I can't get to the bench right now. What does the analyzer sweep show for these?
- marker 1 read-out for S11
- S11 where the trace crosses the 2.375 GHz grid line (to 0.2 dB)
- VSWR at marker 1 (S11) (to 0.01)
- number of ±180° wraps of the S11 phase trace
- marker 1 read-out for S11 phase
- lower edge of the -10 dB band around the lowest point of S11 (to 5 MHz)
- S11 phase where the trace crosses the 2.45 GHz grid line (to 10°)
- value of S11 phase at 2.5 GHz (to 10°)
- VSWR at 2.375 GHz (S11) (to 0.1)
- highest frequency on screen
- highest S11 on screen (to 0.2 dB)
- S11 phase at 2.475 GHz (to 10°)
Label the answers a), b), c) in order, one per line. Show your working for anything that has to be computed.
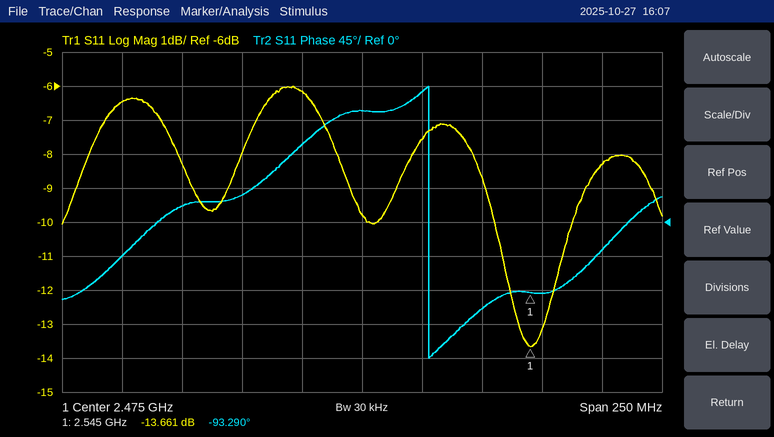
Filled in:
a) -13.661 dB
b) -6.4 dB
c) (1 + 0.2075)/(1 − 0.2075) ≈ 1.52
d) 1
e) -93.290°
f) 2.530 GHz
g) 100°
h) 170°
i) |Γ| = 10^(-6.4/20) = 0.4786; VSWR = (1 + 0.4786)/(1 − 0.4786) ≈ 2.8
j) 2.6 GHz
k) -6.0 dB
l) 150°
